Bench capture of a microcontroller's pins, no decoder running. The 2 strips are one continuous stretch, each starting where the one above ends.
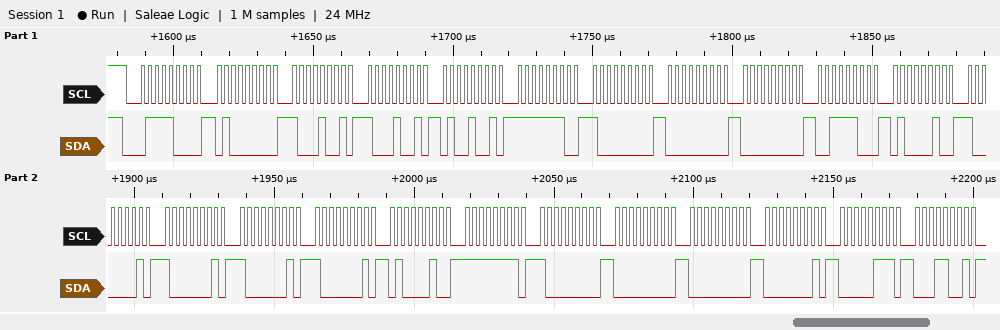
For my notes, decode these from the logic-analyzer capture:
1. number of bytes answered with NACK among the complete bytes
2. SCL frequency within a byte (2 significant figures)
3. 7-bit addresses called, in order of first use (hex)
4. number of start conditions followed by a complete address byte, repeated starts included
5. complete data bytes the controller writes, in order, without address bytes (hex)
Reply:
0
400 kHz
0x3C
1
40 89 89 49 FE 80 00 00 3C 42 81 81 81 81 42 FF 80 00 00 01 07 19
